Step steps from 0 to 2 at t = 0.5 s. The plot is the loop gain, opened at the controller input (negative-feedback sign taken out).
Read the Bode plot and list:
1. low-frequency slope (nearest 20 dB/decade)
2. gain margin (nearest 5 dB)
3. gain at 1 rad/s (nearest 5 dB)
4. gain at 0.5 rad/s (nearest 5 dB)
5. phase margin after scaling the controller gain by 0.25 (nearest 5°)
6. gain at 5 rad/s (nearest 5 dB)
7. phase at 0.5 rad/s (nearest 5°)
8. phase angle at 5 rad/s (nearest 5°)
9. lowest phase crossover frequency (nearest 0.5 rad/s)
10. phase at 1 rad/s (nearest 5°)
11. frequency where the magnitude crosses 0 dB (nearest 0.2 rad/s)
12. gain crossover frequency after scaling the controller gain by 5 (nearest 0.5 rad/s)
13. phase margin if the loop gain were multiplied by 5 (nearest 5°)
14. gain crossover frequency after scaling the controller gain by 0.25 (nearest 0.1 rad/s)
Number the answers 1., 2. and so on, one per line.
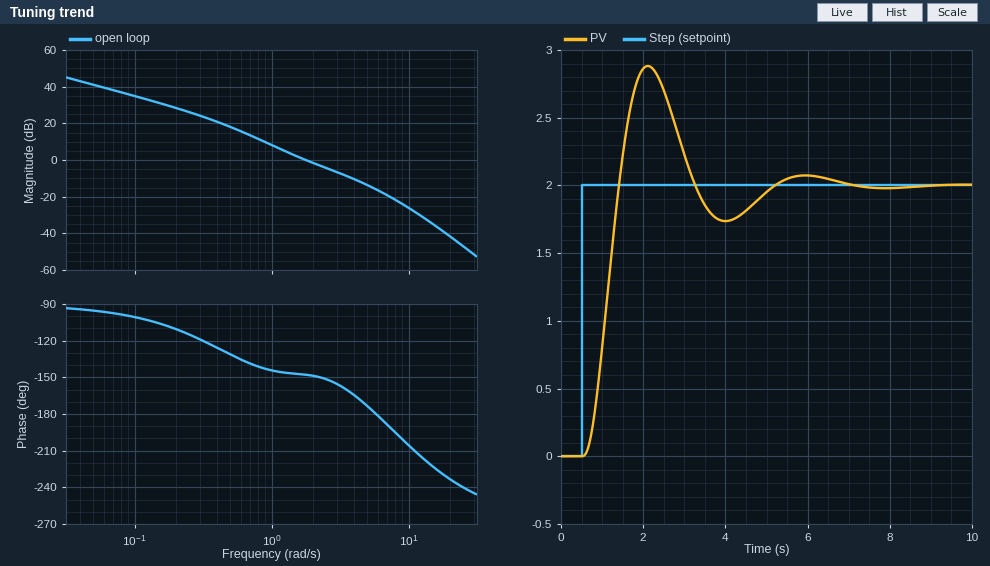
1. -20 dB/decade
2. 15 dB
3. 10 dB
4. 20 dB
5. 40°
6. -15 dB
7. -130°
8. -175°
9. 6.0 rad/s
10. -145°
11. 1.8 rad/s
12. 5.0 rad/s
13. 5°
14. 0.8 rad/s
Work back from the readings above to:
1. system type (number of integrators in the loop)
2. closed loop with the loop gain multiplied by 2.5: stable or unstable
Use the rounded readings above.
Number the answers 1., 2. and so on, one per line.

1. 1
2. stable
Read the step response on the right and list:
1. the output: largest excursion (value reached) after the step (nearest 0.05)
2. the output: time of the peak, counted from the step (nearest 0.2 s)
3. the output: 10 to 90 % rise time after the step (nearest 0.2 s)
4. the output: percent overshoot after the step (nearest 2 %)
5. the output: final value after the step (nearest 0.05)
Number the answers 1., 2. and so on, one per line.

1. 2.90
2. 1.6 s
3. 0.6 s
4. 44 %
5. 2.00
